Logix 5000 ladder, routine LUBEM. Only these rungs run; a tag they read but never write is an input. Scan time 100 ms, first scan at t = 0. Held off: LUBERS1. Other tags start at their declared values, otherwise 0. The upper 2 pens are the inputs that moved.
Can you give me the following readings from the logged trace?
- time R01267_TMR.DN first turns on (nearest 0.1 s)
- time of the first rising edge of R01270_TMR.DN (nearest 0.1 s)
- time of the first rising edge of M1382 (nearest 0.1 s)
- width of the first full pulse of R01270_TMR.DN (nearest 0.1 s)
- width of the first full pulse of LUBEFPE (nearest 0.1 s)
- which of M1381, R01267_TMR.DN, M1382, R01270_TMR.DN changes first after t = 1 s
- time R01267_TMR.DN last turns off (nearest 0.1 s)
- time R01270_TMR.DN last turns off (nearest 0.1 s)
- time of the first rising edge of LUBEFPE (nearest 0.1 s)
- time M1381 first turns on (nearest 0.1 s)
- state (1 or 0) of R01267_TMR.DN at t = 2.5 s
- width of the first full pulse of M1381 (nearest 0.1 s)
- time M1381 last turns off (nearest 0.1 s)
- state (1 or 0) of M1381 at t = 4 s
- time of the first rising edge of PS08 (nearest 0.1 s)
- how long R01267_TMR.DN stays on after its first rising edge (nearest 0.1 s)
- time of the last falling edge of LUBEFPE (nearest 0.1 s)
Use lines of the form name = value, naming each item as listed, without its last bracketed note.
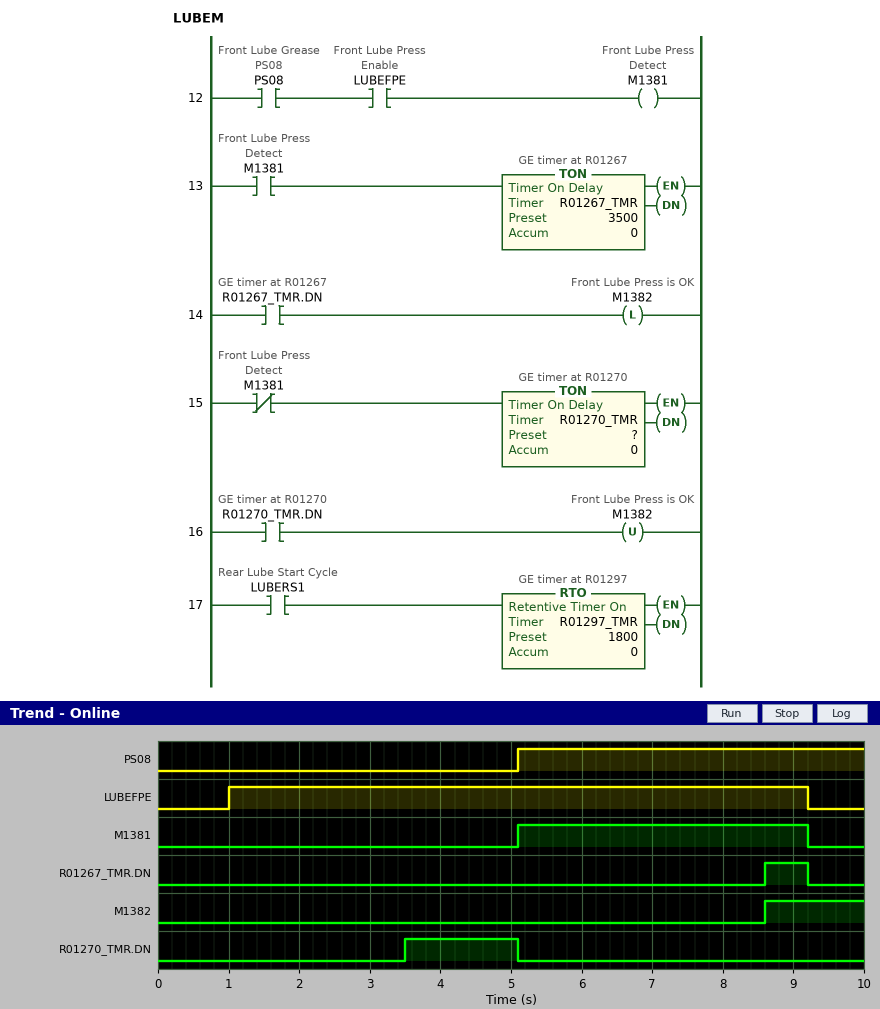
time R01267_TMR.DN first turns on = 8.6 s
time of the first rising edge of R01270_TMR.DN = 3.5 s
time of the first rising edge of M1382 = 8.6 s
width of the first full pulse of R01270_TMR.DN = 1.6 s
width of the first full pulse of LUBEFPE = 8.2 s
which of M1381, R01267_TMR.DN, M1382, R01270_TMR.DN changes first after t = 1 s = R01270_TMR.DN
time R01267_TMR.DN last turns off = 9.2 s
time R01270_TMR.DN last turns off = 5.1 s
time of the first rising edge of LUBEFPE = 1.0 s
time M1381 first turns on = 5.1 s
state (1 or 0) of R01267_TMR.DN at t = 2.5 s = 0
width of the first full pulse of M1381 = 4.1 s
time M1381 last turns off = 9.2 s
state (1 or 0) of M1381 at t = 4 s = 0
time of the first rising edge of PS08 = 5.1 s
how long R01267_TMR.DN stays on after its first rising edge = 0.6 s
time of the last falling edge of LUBEFPE = 9.2 s
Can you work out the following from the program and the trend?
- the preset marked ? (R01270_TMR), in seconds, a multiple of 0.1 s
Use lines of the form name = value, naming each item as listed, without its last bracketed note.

the preset marked ? (R01270_TMR), in seconds, a multiple of 0.1 s = 3.5 s
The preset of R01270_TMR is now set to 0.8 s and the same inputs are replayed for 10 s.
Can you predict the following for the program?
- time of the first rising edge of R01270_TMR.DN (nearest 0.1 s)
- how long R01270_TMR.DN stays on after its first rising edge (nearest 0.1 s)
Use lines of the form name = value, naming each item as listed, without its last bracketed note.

time of the first rising edge of R01270_TMR.DN = 0.8 s
how long R01270_TMR.DN stays on after its first rising edge = 4.3 s
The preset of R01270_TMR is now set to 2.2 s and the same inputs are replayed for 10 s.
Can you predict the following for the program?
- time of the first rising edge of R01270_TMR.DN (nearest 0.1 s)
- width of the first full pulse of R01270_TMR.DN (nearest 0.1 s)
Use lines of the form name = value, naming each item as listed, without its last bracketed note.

time of the first rising edge of R01270_TMR.DN = 2.2 s
width of the first full pulse of R01270_TMR.DN = 2.9 s
